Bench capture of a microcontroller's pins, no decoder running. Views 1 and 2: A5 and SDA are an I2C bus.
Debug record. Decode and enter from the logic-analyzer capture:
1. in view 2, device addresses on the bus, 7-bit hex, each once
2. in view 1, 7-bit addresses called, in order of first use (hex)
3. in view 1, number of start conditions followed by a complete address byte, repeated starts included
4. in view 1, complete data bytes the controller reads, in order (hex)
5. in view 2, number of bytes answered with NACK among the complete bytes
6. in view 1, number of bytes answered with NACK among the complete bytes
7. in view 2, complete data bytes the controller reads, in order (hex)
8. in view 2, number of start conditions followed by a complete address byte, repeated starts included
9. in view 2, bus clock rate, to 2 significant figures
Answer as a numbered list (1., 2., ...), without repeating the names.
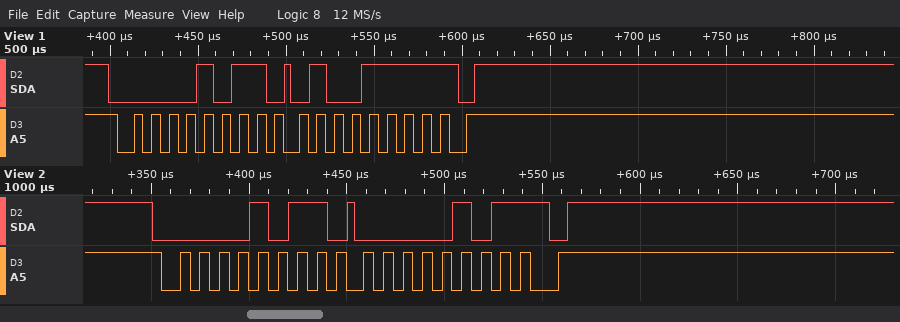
1. 0x05
2. 0x05
3. 1
4. 4F
5. 1
6. 1
7. 05
8. 1
9. 100 kHz
